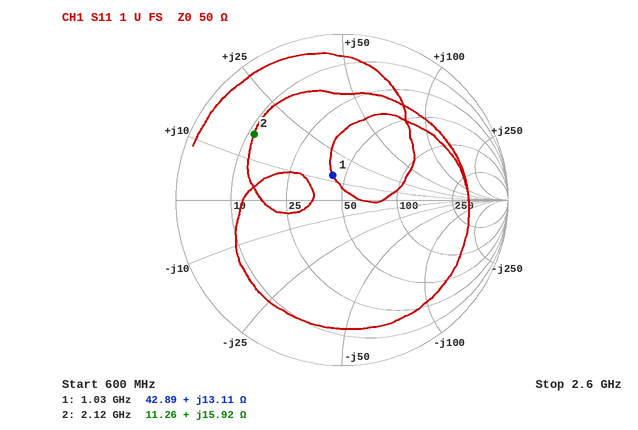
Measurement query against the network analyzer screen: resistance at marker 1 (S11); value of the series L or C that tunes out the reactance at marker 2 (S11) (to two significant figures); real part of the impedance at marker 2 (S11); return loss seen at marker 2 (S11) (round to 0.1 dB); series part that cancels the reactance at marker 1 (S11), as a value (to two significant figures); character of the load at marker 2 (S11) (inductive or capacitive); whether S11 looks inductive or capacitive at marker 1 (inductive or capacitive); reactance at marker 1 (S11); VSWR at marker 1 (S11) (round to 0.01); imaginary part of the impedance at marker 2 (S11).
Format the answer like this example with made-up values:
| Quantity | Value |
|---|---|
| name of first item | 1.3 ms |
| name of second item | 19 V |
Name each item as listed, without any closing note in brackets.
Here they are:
| Quantity | Value |
|---|---|
| resistance at marker 1 | 42.89 Ω |
| value of the series L or C that tunes out the reactance at marker 2 (S11) | 4.7 pF |
| real part of the impedance at marker 2 | 11.26 Ω |
| return loss seen at marker 2 (S11) | 3.6 dB |
| series part that cancels the reactance at marker 1 (S11), as a value | 12 pF |
| character of the load at marker 2 (S11) | inductive |
| whether S11 looks inductive or capacitive at marker 1 | inductive |
| reactance at marker 1 | +13.11 Ω |
| VSWR at marker 1 (S11) | 1.38 |
| imaginary part of the impedance at marker 2 | +15.92 Ω |
